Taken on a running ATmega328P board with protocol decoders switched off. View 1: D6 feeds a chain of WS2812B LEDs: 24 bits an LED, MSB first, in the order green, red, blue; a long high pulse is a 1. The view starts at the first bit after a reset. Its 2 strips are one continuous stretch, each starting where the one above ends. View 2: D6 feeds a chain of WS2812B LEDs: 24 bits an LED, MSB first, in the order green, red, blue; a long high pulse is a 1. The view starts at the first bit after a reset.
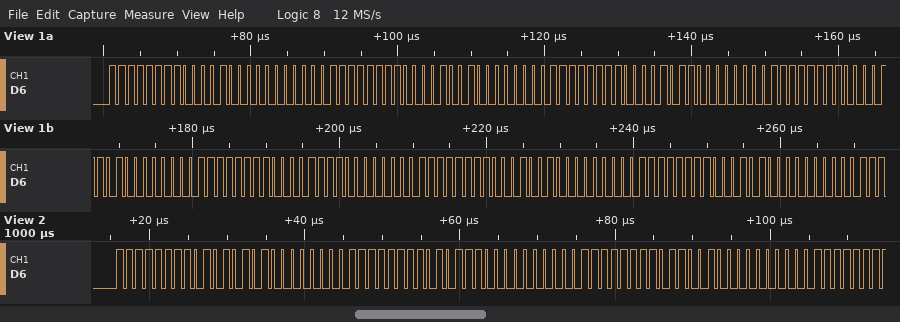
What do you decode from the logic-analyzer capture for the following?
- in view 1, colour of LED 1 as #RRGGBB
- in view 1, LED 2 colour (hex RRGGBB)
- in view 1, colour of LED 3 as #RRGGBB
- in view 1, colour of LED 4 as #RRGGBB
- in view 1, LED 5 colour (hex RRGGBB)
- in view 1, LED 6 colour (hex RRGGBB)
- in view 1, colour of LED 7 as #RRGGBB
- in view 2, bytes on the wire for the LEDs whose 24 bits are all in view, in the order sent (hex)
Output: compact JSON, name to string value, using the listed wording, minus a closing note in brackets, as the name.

{"in view 1, colour of LED 1 as #RRGGBB": "#08FF00", "in view 1, LED 2 colour": "#09FF00", "in view 1, colour of LED 3 as #RRGGBB": "#0BFF00", "in view 1, colour of LED 4 as #RRGGBB": "#0DFF00", "in view 1, LED 5 colour": "#0FFF00", "in view 1, LED 6 colour": "#12FF00", "in view 1, colour of LED 7 as #RRGGBB": "#14FF00", "in view 2, bytes on the wire for the LEDs whose 24 bits are all in view, in the order sent": "FF 55 00 FF 5C 00 FF 64 00"}
